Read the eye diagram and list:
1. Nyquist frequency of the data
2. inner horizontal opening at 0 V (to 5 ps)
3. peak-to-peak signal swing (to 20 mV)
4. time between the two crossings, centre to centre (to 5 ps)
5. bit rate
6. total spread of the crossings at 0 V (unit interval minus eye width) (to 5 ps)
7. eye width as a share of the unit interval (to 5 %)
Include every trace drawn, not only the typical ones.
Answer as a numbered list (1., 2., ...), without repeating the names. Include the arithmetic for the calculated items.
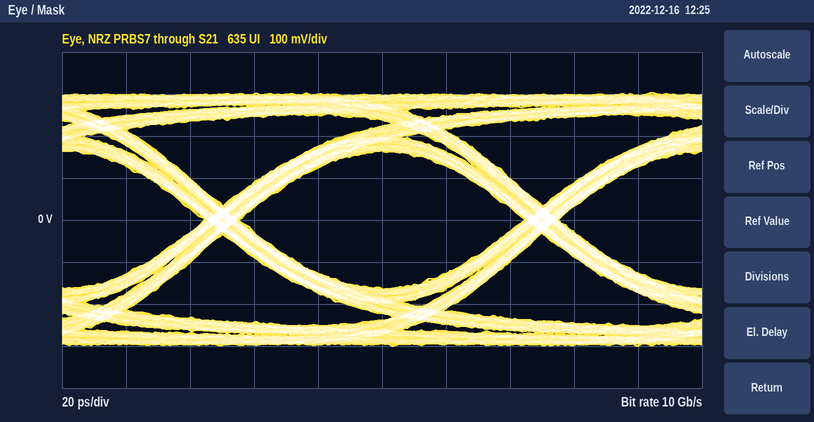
1. 5 GHz
2. 90 ps
3. 600 mV
4. 100 ps
5. 10 Gb/s
6. 10 ps
7. 90 ps / 100 ps ≈ 90 %
